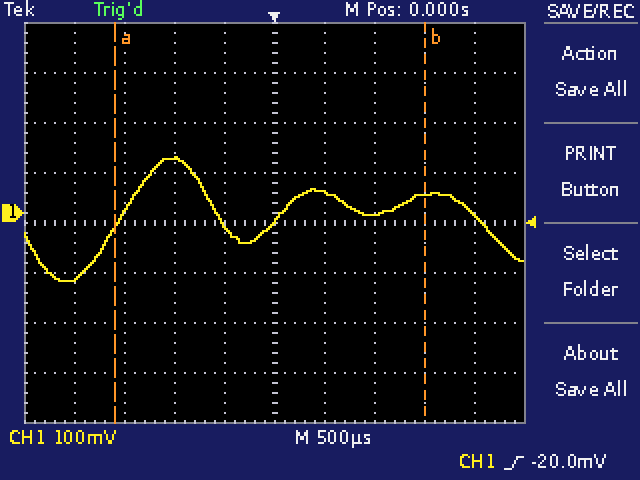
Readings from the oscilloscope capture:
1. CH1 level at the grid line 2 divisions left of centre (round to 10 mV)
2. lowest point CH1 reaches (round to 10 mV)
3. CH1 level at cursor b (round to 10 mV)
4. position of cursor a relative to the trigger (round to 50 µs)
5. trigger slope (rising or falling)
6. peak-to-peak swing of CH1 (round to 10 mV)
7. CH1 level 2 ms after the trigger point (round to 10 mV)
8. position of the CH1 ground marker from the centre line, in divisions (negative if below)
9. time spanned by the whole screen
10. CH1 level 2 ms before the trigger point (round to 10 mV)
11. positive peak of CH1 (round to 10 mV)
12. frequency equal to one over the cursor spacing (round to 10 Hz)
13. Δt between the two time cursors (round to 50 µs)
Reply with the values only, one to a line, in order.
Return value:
110 mV
-140 mV
40 mV
-1.60 ms
rising
250 mV
0 mV
+0.2 div
5 ms
-130 mV
110 mV
320 Hz
3.10 ms
